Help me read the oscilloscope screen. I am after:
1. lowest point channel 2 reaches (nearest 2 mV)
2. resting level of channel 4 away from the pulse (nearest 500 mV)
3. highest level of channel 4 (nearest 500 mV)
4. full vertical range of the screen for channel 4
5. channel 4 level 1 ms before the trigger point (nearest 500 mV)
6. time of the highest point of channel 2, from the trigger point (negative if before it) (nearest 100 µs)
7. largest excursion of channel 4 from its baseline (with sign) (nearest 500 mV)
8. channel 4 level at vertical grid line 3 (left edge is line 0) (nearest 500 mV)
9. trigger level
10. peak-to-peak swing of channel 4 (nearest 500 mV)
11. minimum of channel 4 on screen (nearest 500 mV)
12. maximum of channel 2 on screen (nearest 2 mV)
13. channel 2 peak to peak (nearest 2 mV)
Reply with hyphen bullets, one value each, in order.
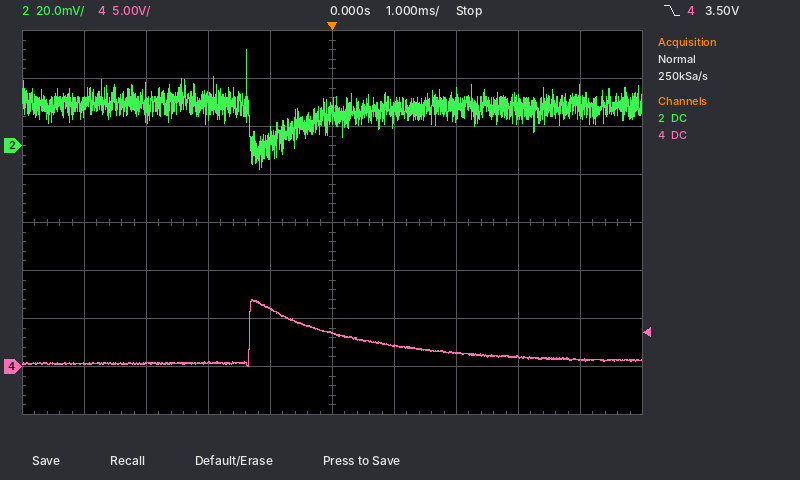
- -10 mV
- 500 mV
- 7.0 V
- 40 V
- 6.0 V
- -1.4 ms
- +6.5 V
- 500 mV
- 3.50 V
- 7.0 V
- 0.0 V
- 40 mV
- 50 mV
